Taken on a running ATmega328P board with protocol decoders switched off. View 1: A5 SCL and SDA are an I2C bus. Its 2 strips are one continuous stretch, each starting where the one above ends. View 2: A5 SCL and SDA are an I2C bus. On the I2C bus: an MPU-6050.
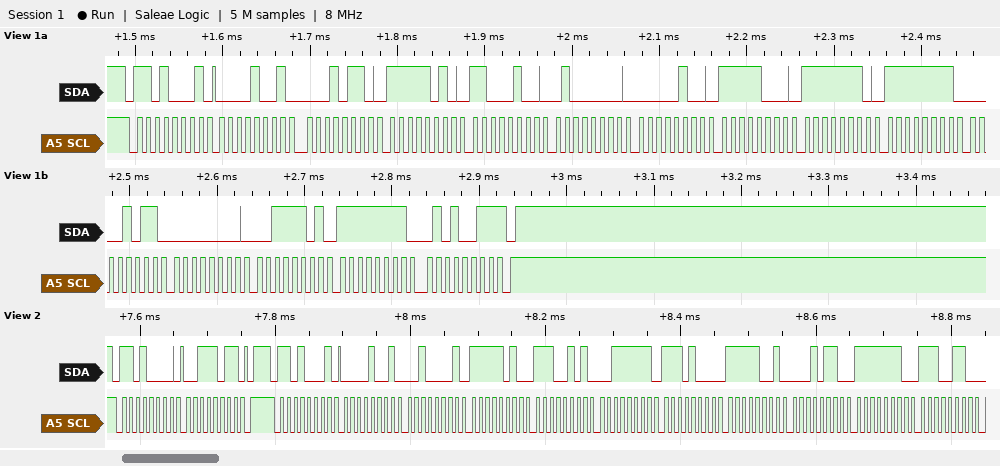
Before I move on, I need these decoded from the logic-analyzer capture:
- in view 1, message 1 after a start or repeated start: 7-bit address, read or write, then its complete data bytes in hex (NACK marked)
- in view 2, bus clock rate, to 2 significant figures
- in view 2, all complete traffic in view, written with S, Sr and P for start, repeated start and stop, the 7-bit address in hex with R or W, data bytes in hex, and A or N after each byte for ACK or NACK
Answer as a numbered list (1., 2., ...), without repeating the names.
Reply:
1. 0x68 read: 09 16 FA C4 40 04 F8 FE FF 0B 00 3D FF 53 NACK
2. 100 kHz
3. S 68W A 3B A P S 68R A 09 A 21 A FA A E5 A 3F A E8 A F9 A 16 A FE A E6 A
